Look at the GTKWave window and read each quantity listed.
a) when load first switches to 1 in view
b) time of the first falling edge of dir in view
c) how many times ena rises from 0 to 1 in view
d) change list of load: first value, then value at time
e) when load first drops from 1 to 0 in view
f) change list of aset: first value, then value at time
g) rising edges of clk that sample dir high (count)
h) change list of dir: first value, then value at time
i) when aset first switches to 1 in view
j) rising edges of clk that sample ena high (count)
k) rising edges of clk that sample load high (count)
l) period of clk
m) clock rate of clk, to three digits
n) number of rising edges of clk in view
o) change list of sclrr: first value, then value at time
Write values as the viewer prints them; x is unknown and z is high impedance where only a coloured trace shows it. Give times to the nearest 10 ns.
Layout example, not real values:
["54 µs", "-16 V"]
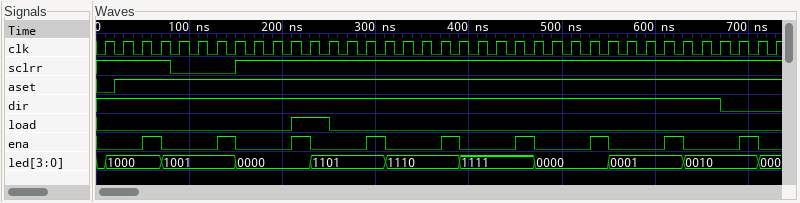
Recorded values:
["210 ns", "670 ns", "9", "0, 1 at 210 ns, 0 at 250 ns", "250 ns", "0, 1 at 20 ns", "34", "1, 0 at 670 ns", "20 ns", "9", "2", "20 ns", "50.0 MHz", "37", "1, 0 at 80 ns, 1 at 150 ns"]
